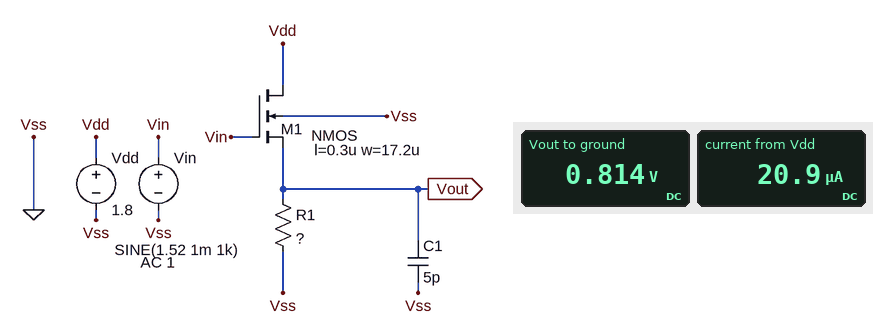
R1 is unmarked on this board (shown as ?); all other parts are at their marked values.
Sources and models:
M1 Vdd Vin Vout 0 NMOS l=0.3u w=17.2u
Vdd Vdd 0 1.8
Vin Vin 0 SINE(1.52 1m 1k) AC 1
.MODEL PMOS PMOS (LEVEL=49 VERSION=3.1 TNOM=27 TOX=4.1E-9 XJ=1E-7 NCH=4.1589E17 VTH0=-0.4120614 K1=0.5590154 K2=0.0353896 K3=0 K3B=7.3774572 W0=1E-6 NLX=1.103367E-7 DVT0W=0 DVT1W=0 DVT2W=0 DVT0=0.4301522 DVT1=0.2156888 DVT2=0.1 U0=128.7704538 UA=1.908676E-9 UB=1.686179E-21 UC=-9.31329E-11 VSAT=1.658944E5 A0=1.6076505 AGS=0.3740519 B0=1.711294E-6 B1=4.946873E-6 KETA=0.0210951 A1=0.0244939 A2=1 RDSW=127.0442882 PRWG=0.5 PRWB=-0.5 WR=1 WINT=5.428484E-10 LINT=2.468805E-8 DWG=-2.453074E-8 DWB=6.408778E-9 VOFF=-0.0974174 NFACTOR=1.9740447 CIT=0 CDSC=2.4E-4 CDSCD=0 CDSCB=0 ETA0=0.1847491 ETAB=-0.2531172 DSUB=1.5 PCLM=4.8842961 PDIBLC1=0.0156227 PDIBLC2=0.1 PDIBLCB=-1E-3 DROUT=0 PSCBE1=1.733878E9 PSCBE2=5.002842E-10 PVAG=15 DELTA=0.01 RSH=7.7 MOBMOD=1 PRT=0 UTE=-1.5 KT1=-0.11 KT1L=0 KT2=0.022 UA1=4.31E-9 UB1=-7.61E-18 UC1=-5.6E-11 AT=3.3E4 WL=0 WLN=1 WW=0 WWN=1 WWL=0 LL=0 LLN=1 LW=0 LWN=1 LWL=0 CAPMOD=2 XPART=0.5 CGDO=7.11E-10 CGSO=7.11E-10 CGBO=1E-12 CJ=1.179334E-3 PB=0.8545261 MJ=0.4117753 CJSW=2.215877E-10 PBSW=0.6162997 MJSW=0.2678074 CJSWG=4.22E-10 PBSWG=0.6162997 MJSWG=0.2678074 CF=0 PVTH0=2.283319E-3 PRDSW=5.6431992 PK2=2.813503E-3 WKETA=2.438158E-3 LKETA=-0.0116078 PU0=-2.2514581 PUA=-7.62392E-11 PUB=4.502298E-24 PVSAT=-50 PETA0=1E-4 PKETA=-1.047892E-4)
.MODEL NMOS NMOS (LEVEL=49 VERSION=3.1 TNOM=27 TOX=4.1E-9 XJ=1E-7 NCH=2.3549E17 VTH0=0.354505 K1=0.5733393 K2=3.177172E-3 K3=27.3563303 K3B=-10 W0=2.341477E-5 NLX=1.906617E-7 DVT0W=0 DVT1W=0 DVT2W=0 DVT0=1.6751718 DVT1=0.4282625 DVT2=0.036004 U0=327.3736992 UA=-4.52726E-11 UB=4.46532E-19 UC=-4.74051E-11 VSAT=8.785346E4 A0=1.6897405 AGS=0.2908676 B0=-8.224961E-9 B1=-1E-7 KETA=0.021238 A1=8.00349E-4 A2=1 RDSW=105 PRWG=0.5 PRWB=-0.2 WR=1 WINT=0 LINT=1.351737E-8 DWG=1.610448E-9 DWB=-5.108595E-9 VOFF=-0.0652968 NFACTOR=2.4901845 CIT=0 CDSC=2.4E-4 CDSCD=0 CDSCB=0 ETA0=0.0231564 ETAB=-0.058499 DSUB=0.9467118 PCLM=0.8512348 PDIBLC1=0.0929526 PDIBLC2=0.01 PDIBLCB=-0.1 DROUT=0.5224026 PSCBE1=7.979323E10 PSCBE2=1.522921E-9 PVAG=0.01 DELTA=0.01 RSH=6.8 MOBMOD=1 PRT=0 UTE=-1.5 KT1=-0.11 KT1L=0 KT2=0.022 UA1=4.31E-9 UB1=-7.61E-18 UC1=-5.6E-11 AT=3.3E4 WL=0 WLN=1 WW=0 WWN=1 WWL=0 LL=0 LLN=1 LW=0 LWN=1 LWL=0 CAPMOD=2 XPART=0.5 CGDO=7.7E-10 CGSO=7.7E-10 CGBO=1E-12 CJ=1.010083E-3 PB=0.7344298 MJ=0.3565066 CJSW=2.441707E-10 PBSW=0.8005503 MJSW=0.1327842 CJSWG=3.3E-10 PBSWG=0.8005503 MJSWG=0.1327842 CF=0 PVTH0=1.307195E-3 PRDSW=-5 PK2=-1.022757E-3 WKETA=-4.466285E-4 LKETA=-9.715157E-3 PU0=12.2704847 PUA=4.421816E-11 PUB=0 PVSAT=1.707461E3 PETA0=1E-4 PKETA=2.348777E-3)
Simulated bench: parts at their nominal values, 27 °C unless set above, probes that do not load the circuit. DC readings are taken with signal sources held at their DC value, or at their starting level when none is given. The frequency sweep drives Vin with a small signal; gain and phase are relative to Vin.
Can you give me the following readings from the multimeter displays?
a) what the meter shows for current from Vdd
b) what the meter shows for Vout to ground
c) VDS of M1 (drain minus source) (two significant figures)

20.9 µA
0.814 V
990 mV
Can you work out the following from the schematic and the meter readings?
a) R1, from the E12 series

39 kΩ
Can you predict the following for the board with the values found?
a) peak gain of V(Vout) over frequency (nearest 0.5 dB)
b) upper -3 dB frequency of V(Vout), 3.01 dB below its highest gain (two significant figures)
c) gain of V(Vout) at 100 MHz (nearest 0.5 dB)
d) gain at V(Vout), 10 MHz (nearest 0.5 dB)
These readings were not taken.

-2.0 dB
19 MHz
-16.5 dB
-3.0 dB
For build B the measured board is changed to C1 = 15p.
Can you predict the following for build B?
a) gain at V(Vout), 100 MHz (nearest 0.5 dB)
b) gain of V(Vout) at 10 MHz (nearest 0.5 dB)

-26.0 dB
-7.5 dB
